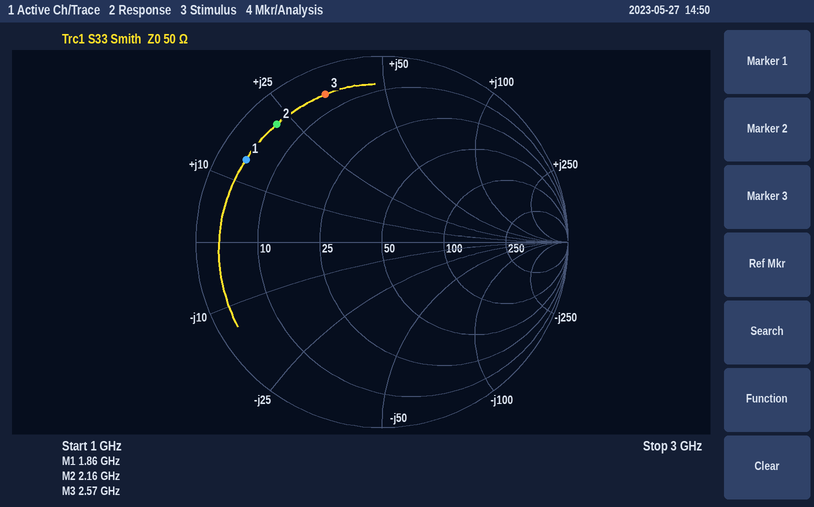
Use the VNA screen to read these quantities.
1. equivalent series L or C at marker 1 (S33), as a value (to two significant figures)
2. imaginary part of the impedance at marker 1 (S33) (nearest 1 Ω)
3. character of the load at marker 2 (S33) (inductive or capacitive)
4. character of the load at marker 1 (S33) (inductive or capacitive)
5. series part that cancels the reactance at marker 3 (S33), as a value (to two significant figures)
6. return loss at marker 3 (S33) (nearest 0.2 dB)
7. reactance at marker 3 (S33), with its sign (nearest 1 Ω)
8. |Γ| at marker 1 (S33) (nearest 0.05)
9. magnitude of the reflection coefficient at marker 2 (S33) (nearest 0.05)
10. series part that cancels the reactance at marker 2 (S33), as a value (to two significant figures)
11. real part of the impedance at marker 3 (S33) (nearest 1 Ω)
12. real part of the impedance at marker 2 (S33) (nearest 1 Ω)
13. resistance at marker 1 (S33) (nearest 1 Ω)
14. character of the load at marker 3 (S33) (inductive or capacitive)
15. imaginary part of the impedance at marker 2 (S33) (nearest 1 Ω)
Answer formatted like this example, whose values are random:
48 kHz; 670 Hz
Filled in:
1.2 nH; +14 Ω; inductive; inductive; 1.8 pF; 1.4 dB; +34 Ω; 0.85; 0.85; 3.3 pF; 6 Ω; 5 Ω; 4 Ω; inductive; +22 Ω
